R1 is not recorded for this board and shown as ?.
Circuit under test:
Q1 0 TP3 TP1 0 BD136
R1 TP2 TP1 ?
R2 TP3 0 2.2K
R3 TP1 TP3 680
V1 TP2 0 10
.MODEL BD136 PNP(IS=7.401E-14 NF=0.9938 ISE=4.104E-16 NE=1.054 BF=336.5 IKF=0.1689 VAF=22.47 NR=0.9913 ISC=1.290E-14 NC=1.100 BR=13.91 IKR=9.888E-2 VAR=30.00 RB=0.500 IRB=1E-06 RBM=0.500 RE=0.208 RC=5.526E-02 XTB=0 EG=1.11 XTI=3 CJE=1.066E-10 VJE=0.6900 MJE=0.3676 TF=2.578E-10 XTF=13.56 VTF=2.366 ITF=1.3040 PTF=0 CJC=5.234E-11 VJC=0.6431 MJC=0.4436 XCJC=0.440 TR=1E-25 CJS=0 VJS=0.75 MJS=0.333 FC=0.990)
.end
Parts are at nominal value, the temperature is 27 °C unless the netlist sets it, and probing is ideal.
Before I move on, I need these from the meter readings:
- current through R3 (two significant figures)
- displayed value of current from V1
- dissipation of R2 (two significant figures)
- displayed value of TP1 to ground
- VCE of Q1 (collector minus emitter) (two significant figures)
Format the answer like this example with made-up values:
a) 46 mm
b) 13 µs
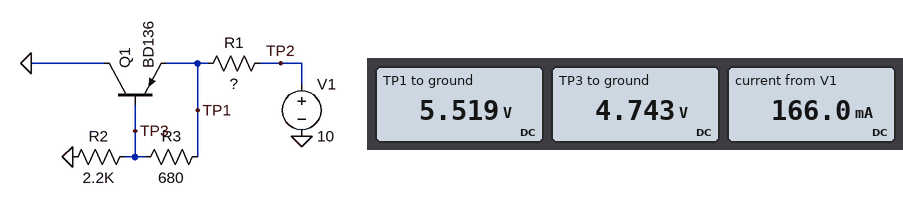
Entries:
a) 1.1 mA
b) 166.0 mA
c) 10 mW
d) 5.519 V
e) -5.5 V
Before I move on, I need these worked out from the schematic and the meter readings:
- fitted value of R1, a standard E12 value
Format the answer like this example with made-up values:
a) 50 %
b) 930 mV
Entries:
a) 27 Ω
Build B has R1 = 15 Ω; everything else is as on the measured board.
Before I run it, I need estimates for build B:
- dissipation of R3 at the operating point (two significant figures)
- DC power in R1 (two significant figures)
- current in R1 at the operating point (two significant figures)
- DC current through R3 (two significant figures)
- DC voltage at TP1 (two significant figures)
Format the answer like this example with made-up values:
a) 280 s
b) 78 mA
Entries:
a) 940 µW
b) 750 mW
c) 220 mA
d) 1.2 mA
e) 6.6 V
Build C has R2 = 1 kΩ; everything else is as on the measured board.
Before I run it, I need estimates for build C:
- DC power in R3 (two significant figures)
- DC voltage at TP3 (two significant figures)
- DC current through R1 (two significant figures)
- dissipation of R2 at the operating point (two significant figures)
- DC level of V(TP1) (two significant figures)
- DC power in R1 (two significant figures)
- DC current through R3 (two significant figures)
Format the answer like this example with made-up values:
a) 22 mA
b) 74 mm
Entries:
a) 950 µW
b) 3.0 V
c) 230 mA
d) 9.0 mW
e) 3.8 V
f) 1.4 W
g) 1.2 mA
